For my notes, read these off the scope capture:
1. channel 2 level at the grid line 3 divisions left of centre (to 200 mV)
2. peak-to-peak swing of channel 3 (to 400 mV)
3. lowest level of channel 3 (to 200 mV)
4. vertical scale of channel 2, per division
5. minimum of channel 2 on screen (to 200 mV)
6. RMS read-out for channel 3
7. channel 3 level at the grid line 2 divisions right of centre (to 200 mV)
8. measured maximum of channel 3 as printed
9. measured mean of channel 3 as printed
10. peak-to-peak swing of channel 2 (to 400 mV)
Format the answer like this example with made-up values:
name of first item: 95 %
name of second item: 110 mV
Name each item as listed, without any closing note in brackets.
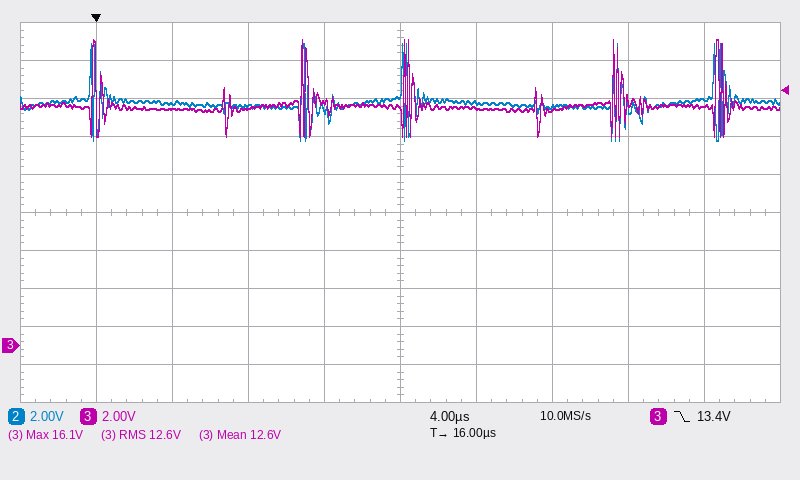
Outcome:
channel 2 level at the grid line 3 divisions left of centre: 12.8 V
peak-to-peak swing of channel 3: 5.2 V
lowest level of channel 3: 11.0 V
vertical scale of channel 2, per division: 2 V
minimum of channel 2 on screen: 10.8 V
RMS read-out for channel 3: 12.6 V
channel 3 level at the grid line 2 divisions right of centre: 12.4 V
measured maximum of channel 3 as printed: 16.1 V
measured mean of channel 3 as printed: 12.6 V
peak-to-peak swing of channel 2: 5.2 V
